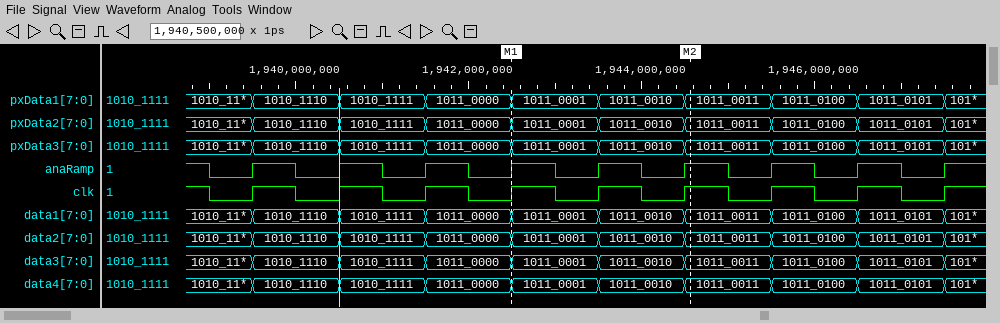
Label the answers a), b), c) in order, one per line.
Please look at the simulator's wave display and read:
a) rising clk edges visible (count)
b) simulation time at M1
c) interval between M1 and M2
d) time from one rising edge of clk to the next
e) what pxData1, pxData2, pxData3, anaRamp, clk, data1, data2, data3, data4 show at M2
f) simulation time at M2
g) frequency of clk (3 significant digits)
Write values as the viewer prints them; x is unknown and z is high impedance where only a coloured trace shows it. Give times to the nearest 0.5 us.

a) 9
b) 1942.5 us
c) 2 us
d) 1 us
e) pxData1=1011_0011, pxData2=1011_0011, pxData3=1011_0011, anaRamp=1, clk=1, data1=1011_0011, data2=1011_0011, data3=1011_0011, data4=1011_0011
f) 1944.5 us
g) 1.00 MHz
